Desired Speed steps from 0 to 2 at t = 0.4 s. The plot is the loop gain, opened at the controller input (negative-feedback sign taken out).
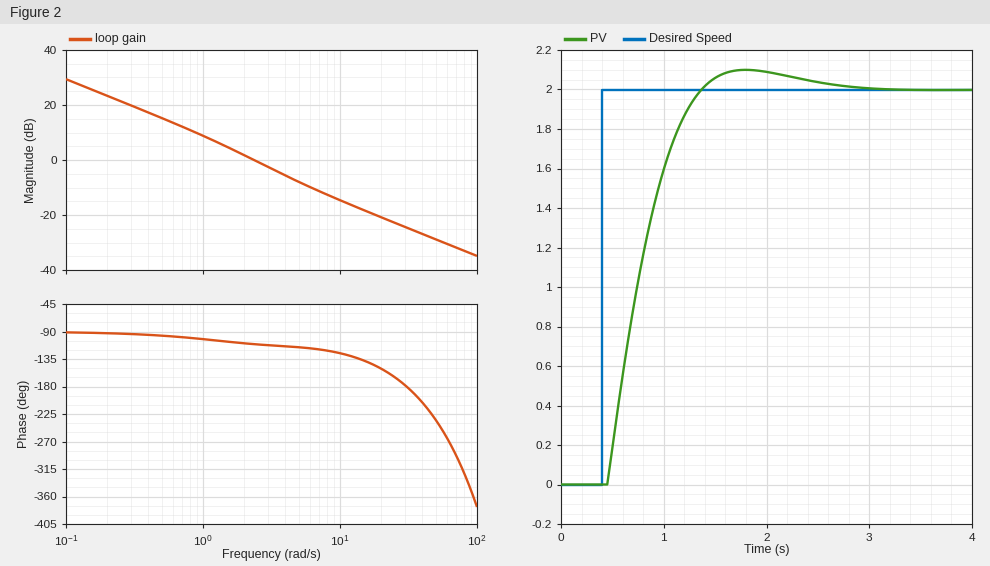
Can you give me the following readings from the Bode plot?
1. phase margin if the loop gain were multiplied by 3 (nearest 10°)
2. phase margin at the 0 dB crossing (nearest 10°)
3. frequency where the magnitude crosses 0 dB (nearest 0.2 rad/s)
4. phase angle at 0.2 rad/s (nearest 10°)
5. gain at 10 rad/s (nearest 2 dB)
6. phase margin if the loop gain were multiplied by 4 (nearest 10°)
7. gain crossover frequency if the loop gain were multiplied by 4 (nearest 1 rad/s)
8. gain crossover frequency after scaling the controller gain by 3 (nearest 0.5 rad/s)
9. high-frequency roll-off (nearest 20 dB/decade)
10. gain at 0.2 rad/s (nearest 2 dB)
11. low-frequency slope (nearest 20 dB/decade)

60°
70°
2.4 rad/s
-90°
-14 dB
60°
8 rad/s
6.0 rad/s
-20 dB/decade
24 dB
-20 dB/decade
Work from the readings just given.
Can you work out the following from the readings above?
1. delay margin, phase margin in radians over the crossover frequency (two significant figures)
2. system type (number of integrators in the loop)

0.51 s
1
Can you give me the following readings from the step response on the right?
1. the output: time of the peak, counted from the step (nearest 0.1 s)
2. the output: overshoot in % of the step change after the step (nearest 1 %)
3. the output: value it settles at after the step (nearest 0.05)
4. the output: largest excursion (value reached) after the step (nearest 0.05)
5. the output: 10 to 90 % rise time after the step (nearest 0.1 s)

1.4 s
5 %
2.00
2.10
0.6 s
